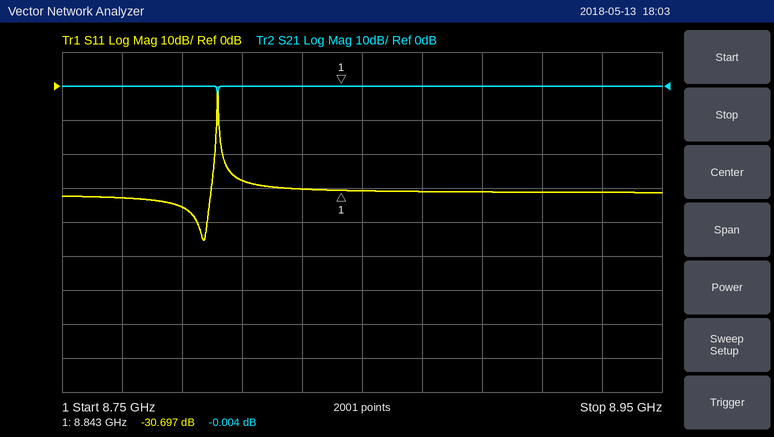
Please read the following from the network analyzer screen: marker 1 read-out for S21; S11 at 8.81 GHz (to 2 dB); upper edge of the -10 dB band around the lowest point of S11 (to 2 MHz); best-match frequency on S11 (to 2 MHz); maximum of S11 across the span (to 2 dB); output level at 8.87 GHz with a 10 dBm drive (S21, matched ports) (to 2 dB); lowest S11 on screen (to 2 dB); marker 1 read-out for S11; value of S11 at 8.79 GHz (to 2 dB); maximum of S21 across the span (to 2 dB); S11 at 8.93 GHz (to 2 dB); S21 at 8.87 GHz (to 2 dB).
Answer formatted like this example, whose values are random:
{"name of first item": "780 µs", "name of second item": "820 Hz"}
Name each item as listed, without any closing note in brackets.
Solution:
{"marker 1 read-out for S21": "-0.004 dB", "S11 at 8.81 GHz": "-28 dB", "upper edge of the -10 dB band around the lowest point of S11": "8.802 GHz", "best-match frequency on S11": "8.798 GHz", "maximum of S11 across the span": "-2 dB", "output level at 8.87 GHz with a 10 dBm drive (S21, matched ports)": "10 dBm", "lowest S11 on screen": "-46 dB", "marker 1 read-out for S11": "-30.697 dB", "value of S11 at 8.79 GHz": "-36 dB", "maximum of S21 across the span": "0 dB", "S11 at 8.93 GHz": "-32 dB", "S21 at 8.87 GHz": "0 dB"}
